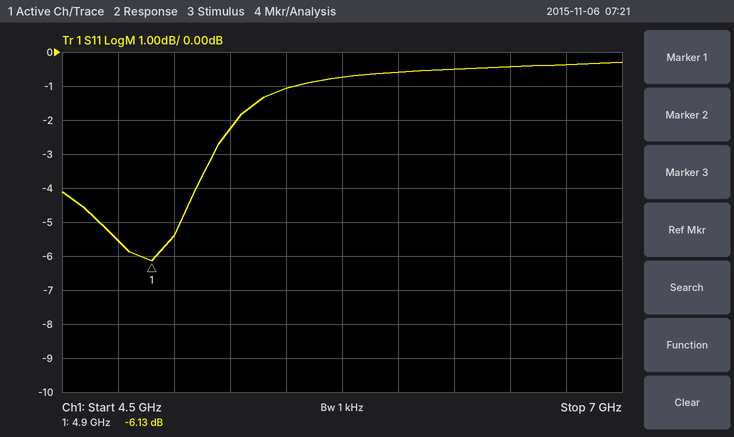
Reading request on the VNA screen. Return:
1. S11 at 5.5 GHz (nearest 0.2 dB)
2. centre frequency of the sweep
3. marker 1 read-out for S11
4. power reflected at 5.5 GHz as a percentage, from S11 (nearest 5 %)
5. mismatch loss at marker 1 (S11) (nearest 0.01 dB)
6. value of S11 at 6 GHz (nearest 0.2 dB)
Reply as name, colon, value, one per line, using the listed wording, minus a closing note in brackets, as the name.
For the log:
S11 at 5.5 GHz: -1.0 dB
centre frequency of the sweep: 5.75 GHz
marker 1 read-out for S11: -6.13 dB
power reflected at 5.5 GHz as a percentage, from S11: 80 %
mismatch loss at marker 1 (S11): 1.21 dB
value of S11 at 6 GHz: -0.6 dB
